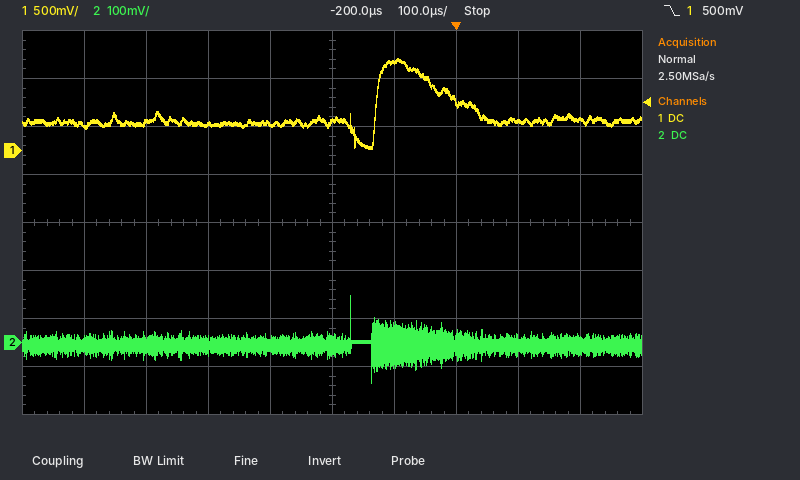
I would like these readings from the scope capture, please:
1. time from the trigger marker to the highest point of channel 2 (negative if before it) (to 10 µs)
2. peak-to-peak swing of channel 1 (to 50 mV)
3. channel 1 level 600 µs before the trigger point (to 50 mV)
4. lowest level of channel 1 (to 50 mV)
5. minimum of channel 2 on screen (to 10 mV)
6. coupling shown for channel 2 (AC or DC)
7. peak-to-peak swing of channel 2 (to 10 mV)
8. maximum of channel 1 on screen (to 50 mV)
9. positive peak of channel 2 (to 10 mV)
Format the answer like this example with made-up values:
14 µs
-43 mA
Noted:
-170 µs
950 mV
250 mV
0 mV
-80 mV
DC
180 mV
950 mV
100 mV
